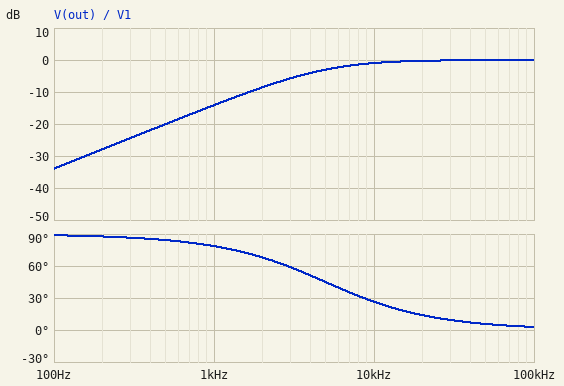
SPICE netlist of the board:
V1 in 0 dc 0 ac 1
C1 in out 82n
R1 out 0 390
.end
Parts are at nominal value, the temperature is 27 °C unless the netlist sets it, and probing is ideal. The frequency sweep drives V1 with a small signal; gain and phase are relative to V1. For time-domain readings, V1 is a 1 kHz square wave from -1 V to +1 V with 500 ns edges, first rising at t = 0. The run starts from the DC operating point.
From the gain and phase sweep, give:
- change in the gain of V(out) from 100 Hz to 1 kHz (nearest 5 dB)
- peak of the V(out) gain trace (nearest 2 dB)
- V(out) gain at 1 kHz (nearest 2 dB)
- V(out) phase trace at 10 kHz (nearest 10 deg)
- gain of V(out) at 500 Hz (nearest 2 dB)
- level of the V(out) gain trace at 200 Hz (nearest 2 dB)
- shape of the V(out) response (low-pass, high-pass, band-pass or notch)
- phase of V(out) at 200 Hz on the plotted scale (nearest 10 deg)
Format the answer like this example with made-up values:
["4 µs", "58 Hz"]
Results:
["20 dB", "0 dB", "-14 dB", "30 deg", "-20 dB", "-28 dB", "high-pass", "90 deg"]
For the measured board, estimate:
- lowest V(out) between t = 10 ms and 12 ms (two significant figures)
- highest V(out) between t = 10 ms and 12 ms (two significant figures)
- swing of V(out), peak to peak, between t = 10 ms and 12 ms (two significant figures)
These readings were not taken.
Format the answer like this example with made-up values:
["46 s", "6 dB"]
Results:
["-2.0 V", "2.0 V", "4.0 V"]
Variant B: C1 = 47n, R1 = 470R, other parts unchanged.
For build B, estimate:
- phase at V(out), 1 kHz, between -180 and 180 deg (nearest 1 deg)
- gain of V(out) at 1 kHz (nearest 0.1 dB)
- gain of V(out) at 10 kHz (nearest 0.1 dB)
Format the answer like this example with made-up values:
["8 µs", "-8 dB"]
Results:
["82 deg", "-17.2 dB", "-1.8 dB"]
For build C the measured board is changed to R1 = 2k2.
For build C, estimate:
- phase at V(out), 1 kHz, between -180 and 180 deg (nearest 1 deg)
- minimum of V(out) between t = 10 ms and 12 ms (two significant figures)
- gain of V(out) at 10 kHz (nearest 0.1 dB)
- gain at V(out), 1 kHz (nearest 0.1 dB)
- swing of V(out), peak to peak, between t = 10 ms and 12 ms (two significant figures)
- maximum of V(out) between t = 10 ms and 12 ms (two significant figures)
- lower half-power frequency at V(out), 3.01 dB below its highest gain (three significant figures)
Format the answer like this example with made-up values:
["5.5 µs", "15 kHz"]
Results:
["41 deg", "-1.9 V", "0 dB", "-2.5 dB", "3.8 V", "1.9 V", "882 Hz"]
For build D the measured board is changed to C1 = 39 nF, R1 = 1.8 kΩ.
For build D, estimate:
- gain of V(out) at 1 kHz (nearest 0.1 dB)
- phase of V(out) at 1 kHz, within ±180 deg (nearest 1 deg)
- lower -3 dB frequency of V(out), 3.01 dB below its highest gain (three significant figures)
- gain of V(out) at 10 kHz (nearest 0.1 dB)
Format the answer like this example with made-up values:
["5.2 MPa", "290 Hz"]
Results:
["-7.9 dB", "66 deg", "2.27 kHz", "-0.2 dB"]
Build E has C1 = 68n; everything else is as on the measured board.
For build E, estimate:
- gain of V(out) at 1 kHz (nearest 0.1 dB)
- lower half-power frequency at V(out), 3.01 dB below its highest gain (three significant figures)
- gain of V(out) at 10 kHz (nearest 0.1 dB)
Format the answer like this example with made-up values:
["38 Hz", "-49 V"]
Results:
["-15.7 dB", "6.00 kHz", "-1.3 dB"]
